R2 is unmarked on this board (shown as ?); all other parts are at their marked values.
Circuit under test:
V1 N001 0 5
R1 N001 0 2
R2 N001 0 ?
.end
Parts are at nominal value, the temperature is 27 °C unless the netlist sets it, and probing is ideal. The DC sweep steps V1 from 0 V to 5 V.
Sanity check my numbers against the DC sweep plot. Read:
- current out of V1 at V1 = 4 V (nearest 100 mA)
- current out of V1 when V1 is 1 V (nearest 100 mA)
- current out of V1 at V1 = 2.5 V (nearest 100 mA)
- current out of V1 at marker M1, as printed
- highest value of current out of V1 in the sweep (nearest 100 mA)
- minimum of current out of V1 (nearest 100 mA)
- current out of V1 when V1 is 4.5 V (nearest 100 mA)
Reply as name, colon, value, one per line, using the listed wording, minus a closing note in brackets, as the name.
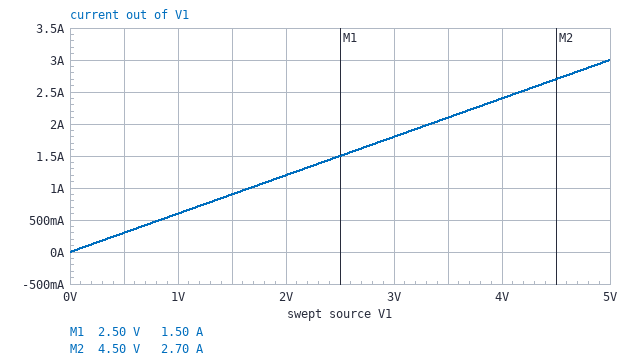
current out of V1 at V1 = 4 V: 2.4 A
current out of V1 when V1 is 1 V: 600 mA
current out of V1 at V1 = 2.5 V: 1.5 A
current out of V1 at marker M1, as printed: 1.50 A
highest value of current out of V1 in the sweep: 3.0 A
minimum of current out of V1: 0 A
current out of V1 when V1 is 4.5 V: 2.7 A
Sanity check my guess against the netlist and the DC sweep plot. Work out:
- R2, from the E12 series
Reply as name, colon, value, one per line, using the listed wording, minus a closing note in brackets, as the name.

R2, from the E12 series: 10 Ω
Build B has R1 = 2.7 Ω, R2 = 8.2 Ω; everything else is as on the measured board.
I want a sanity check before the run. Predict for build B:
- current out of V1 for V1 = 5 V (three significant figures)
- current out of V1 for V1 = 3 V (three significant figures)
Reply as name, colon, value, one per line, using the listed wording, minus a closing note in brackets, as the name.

current out of V1 for V1 = 5 V: 2.46 A
current out of V1 for V1 = 3 V: 1.48 A
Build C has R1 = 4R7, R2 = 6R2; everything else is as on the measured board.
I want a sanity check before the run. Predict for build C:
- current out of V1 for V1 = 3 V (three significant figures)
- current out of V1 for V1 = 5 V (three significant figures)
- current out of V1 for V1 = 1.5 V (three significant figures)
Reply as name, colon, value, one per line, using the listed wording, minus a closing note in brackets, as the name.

current out of V1 for V1 = 3 V: 1.12 A
current out of V1 for V1 = 5 V: 1.87 A
current out of V1 for V1 = 1.5 V: 561 mA
